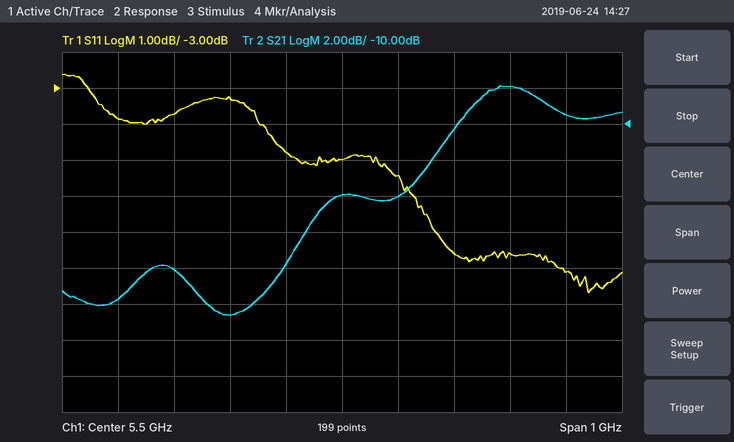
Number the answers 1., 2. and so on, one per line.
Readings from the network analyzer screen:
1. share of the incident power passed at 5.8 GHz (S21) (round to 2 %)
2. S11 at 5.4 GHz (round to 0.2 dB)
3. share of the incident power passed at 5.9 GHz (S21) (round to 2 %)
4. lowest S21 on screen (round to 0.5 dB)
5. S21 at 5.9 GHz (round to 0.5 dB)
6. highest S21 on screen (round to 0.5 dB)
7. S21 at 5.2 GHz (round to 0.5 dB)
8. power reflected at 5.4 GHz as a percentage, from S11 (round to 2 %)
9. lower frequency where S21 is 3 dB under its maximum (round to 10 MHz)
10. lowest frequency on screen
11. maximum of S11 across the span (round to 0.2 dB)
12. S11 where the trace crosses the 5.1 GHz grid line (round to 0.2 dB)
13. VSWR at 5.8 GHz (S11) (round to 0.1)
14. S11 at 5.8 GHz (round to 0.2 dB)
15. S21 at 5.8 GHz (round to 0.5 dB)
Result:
1. 16 %
2. -4.8 dB
3. 12 %
4. -20.5 dB
5. -9.5 dB
6. -8.0 dB
7. -18.0 dB
8. 34 %
9. 5.69 GHz
10. 5 GHz
11. -2.6 dB
12. -3.8 dB
13. 2.4
14. -7.6 dB
15. -8.0 dB
